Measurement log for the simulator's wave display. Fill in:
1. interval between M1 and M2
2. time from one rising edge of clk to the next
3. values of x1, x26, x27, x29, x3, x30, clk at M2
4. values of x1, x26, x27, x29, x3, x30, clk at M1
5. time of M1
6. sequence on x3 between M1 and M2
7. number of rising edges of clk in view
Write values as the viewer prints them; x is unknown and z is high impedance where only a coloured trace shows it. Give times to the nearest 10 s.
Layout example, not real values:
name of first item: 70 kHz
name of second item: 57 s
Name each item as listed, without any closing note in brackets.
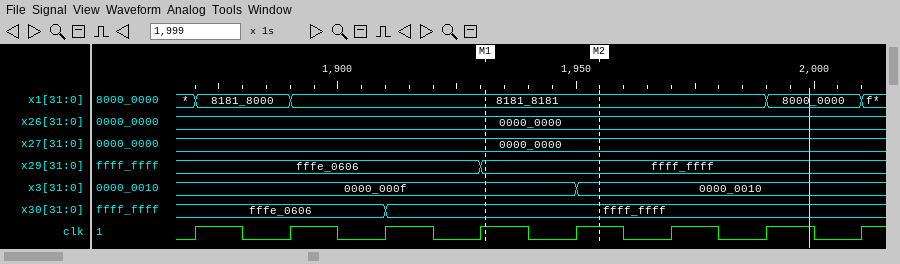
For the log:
interval between M1 and M2: 20 s
time from one rising edge of clk to the next: 20 s
values of x1, x26, x27, x29, x3, x30, clk at M2: x1=8181_8181, x26=0000_0000, x27=0000_0000, x29=ffff_ffff, x3=0000_0010, x30=ffff_ffff, clk=1
values of x1, x26, x27, x29, x3, x30, clk at M1: x1=8181_8181, x26=0000_0000, x27=0000_0000, x29=ffff_ffff, x3=0000_000f, x30=ffff_ffff, clk=1
time of M1: 1930 s
sequence on x3 between M1 and M2: 0000_000f, 0000_0010
number of rising edges of clk in view: 8
